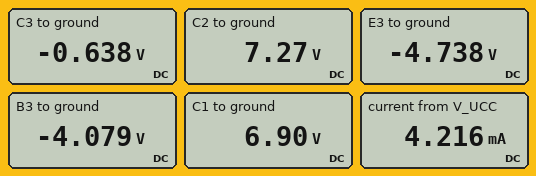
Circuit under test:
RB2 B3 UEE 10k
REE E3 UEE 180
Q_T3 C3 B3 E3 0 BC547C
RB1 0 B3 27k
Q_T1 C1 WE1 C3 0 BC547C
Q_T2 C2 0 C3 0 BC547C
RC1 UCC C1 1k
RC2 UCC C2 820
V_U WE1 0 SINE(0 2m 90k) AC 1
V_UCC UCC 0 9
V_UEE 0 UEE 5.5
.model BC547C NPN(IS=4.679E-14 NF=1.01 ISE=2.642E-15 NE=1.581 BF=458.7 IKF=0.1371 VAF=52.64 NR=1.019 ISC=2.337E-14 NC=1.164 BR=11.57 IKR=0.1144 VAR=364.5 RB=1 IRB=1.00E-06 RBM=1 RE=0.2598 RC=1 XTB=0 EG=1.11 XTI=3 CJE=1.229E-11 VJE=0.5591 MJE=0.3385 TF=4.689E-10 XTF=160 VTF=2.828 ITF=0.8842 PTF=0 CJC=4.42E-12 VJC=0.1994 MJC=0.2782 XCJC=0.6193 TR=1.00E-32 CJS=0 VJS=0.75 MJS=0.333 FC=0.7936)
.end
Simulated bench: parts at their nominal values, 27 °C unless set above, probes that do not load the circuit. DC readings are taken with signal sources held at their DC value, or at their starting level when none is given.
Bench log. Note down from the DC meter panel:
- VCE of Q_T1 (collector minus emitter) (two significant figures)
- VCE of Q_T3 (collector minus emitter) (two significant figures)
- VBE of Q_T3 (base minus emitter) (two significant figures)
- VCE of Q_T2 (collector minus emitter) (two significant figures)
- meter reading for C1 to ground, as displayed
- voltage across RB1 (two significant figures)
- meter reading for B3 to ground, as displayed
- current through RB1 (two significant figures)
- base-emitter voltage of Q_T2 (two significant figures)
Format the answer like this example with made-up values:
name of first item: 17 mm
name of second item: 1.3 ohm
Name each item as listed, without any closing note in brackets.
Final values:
VCE of Q_T1 (collector minus emitter): 7.5 V
VCE of Q_T3 (collector minus emitter): 4.1 V
VBE of Q_T3 (base minus emitter): 660 mV
VCE of Q_T2 (collector minus emitter): 7.9 V
meter reading for C1 to ground, as displayed: 6.90 V
voltage across RB1: 4.1 V
meter reading for B3 to ground, as displayed: -4.079 V
current through RB1: 150 µA
base-emitter voltage of Q_T2: 640 mV
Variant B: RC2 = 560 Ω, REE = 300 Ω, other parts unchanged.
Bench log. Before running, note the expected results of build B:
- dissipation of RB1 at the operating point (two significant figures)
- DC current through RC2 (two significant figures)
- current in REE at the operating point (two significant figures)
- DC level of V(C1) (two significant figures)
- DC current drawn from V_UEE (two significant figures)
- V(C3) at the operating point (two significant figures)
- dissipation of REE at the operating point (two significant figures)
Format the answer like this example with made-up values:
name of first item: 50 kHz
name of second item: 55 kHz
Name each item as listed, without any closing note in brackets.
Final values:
dissipation of RB1 at the operating point: 610 µW
DC current through RC2: 1.3 mA
current in REE at the operating point: 2.7 mA
DC level of V(C1): 7.7 V
DC current drawn from V_UEE: 2.8 mA
V(C3) at the operating point: -630 mV
dissipation of REE at the operating point: 2.1 mW
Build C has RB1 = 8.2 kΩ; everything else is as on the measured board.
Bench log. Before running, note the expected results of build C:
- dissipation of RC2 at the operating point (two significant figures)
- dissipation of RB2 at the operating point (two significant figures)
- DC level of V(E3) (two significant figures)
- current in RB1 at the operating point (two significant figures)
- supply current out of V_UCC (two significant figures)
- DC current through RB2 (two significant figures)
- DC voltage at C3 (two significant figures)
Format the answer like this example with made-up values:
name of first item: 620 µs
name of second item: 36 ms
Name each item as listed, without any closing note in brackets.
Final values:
dissipation of RC2 at the operating point: 31 mW
dissipation of RB2 at the operating point: 840 µW
DC level of V(E3): -3.3 V
current in RB1 at the operating point: 320 µA
supply current out of V_UCC: 12 mA
DC current through RB2: 290 µA
DC voltage at C3: -670 mV
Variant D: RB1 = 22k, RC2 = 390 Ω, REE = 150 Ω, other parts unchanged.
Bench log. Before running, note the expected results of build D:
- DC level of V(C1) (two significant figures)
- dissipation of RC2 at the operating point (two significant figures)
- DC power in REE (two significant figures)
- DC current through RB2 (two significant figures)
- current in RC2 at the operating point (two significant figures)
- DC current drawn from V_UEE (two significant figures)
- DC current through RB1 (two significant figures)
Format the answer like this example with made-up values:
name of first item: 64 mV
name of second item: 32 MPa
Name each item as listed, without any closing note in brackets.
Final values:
DC level of V(C1): 5.9 V
dissipation of RC2 at the operating point: 4.0 mW
DC power in REE: 6.1 mW
DC current through RB2: 160 µA
current in RC2 at the operating point: 3.2 mA
DC current drawn from V_UEE: 6.5 mA
DC current through RB1: 180 µA
